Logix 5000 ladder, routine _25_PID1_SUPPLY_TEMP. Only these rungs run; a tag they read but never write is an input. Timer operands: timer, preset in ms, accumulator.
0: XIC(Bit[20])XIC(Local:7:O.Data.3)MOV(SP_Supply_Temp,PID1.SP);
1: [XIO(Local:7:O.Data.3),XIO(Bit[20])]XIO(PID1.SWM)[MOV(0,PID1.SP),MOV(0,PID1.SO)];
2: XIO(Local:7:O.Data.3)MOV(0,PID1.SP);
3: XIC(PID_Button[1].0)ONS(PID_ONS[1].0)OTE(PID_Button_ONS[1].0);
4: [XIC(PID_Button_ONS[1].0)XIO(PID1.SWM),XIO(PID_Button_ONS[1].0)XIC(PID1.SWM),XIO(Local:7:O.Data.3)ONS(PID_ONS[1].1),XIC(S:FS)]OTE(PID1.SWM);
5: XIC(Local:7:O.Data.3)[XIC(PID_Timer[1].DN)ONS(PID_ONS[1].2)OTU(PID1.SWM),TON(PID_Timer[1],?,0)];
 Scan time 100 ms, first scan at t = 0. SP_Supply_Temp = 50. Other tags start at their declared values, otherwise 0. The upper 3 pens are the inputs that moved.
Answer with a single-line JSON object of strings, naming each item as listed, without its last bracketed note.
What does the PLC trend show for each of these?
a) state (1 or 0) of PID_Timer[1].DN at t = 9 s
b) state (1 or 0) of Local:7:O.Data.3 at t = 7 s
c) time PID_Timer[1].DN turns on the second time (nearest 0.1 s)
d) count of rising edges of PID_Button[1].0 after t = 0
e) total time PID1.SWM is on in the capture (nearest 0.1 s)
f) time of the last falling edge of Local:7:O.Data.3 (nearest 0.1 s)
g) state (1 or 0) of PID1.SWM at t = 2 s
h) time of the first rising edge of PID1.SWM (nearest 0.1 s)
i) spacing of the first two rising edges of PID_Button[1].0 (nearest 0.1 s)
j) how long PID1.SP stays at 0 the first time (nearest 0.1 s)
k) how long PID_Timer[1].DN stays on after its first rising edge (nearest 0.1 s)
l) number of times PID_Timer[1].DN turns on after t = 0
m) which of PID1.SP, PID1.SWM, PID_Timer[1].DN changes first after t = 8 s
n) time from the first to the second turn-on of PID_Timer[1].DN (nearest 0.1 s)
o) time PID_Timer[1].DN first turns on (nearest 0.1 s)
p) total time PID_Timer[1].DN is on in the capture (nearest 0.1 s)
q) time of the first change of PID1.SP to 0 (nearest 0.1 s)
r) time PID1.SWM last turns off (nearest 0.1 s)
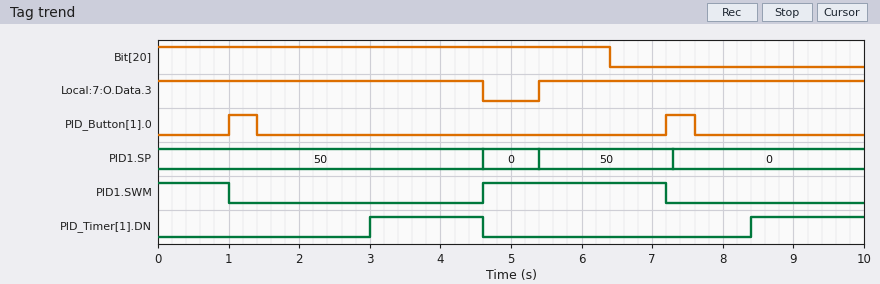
{"state (1 or 0) of PID_Timer[1].DN at t = 9 s": "1", "state (1 or 0) of Local:7:O.Data.3 at t = 7 s": "1", "time PID_Timer[1].DN turns on the second time": "8.4 s", "count of rising edges of PID_Button[1].0 after t = 0": "2", "total time PID1.SWM is on in the capture": "3.6 s", "time of the last falling edge of Local:7:O.Data.3": "4.6 s", "state (1 or 0) of PID1.SWM at t = 2 s": "0", "time of the first rising edge of PID1.SWM": "4.6 s", "spacing of the first two rising edges of PID_Button[1].0": "6.2 s", "how long PID1.SP stays at 0 the first time": "0.8 s", "how long PID_Timer[1].DN stays on after its first rising edge": "1.6 s", "number of times PID_Timer[1].DN turns on after t = 0": "2", "which of PID1.SP, PID1.SWM, PID_Timer[1].DN changes first after t = 8 s": "PID_Timer[1].DN", "time from the first to the second turn-on of PID_Timer[1].DN": "5.4 s", "time PID_Timer[1].DN first turns on": "3.0 s", "total time PID_Timer[1].DN is on in the capture": "3.2 s", "time of the first change of PID1.SP to 0": "4.6 s", "time PID1.SWM last turns off": "7.2 s"}
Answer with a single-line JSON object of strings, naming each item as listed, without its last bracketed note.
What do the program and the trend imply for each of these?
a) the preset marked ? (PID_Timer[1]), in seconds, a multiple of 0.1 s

{"the preset marked ? (PID_Timer[1]), in seconds, a multiple of 0.1 s": "3.0 s"}
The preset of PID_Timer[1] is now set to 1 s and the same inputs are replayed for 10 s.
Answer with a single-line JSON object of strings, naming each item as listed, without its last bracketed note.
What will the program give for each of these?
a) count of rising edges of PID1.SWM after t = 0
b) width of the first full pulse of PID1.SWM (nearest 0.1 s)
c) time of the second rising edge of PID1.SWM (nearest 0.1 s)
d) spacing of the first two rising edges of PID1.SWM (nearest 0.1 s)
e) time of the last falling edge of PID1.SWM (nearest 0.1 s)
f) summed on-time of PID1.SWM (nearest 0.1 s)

{"count of rising edges of PID1.SWM after t = 0": "2", "width of the first full pulse of PID1.SWM": "1.9 s", "time of the second rising edge of PID1.SWM": "7.2 s", "spacing of the first two rising edges of PID1.SWM": "2.6 s", "time of the last falling edge of PID1.SWM": "6.5 s", "summed on-time of PID1.SWM": "5.7 s"}
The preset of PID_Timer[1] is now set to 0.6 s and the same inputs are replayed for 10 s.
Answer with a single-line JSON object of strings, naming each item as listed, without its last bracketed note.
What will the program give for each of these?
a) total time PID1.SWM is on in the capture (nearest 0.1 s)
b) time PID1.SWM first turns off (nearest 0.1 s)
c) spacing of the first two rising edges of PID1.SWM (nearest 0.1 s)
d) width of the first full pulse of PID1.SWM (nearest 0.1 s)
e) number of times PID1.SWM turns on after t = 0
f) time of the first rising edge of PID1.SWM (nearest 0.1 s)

{"total time PID1.SWM is on in the capture": "8.6 s", "time PID1.SWM first turns off": "0.7 s", "spacing of the first two rising edges of PID1.SWM": "6.2 s", "width of the first full pulse of PID1.SWM": "5.1 s", "number of times PID1.SWM turns on after t = 0": "2", "time of the first rising edge of PID1.SWM": "1.0 s"}
